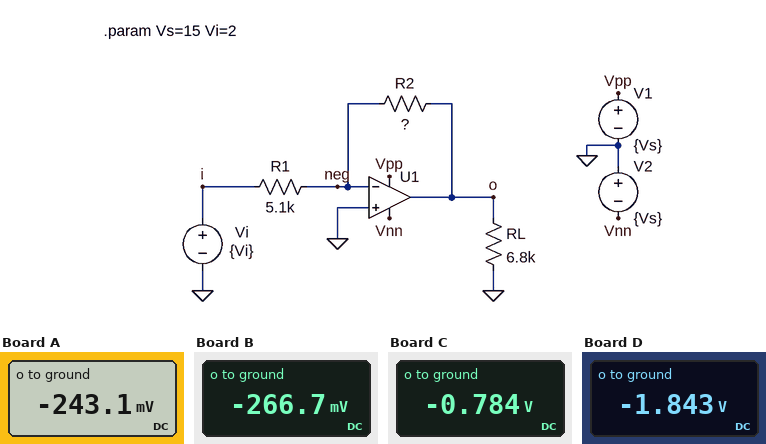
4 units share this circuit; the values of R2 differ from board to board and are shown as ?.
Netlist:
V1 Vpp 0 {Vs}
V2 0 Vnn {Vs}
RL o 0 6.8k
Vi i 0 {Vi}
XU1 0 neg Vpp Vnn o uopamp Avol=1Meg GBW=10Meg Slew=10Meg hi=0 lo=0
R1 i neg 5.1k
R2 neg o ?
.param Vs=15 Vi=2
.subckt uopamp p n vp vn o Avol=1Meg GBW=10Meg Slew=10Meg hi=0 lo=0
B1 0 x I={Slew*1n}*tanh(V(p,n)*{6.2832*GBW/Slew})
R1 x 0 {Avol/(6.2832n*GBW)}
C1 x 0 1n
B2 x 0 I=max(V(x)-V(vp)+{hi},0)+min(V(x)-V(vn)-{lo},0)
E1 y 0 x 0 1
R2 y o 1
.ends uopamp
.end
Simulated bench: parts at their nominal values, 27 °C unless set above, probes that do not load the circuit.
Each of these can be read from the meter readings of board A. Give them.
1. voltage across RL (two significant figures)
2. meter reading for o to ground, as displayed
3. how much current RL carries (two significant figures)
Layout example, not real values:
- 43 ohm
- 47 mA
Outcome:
- 240 mV
- -243.1 mV
- 36 µA
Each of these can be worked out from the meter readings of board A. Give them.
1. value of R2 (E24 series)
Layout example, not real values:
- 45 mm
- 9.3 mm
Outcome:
- 620 Ω
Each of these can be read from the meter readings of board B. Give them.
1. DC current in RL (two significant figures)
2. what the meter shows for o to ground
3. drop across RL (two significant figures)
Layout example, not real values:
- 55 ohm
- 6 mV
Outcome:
- 39 µA
- -266.7 mV
- 270 mV
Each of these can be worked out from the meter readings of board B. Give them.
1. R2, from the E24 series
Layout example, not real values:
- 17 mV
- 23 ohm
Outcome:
- 680 Ω
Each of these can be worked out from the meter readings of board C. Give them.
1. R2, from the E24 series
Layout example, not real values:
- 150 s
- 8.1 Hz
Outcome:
- 2 kΩ
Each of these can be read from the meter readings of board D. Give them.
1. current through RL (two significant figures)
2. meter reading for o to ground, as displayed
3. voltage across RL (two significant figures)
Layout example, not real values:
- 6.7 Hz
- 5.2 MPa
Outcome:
- 270 µA
- -1.843 V
- 1.8 V
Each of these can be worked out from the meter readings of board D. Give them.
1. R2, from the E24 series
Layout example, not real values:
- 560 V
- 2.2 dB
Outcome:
- 4.7 kΩ
